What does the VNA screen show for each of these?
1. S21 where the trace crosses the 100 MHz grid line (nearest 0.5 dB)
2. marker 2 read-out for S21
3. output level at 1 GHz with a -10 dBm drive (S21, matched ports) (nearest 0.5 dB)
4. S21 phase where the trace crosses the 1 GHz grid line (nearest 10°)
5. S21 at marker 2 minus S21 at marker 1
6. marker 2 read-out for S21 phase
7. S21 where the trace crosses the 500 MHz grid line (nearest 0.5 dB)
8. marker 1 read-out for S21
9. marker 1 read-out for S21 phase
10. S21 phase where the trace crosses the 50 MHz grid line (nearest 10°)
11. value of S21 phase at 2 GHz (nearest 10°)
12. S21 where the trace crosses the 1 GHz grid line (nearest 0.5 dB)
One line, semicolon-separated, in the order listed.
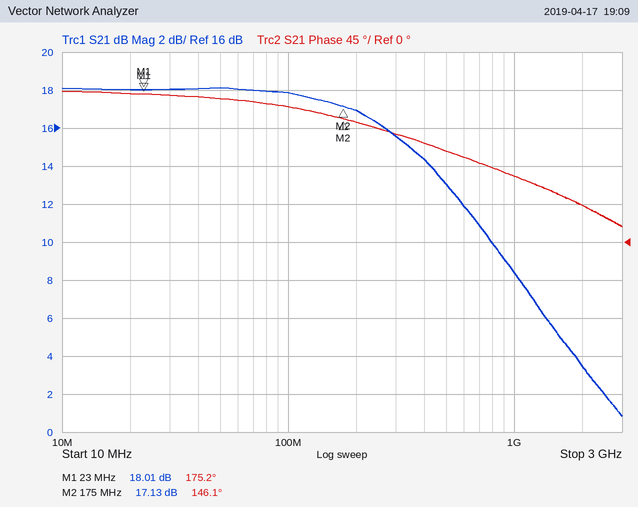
18.0 dB; 17.13 dB; -1.5 dBm; 80°; -0.88 dB; 146.1°; 13.0 dB; 18.01 dB; 175.2°; 170°; 40°; 8.5 dB
